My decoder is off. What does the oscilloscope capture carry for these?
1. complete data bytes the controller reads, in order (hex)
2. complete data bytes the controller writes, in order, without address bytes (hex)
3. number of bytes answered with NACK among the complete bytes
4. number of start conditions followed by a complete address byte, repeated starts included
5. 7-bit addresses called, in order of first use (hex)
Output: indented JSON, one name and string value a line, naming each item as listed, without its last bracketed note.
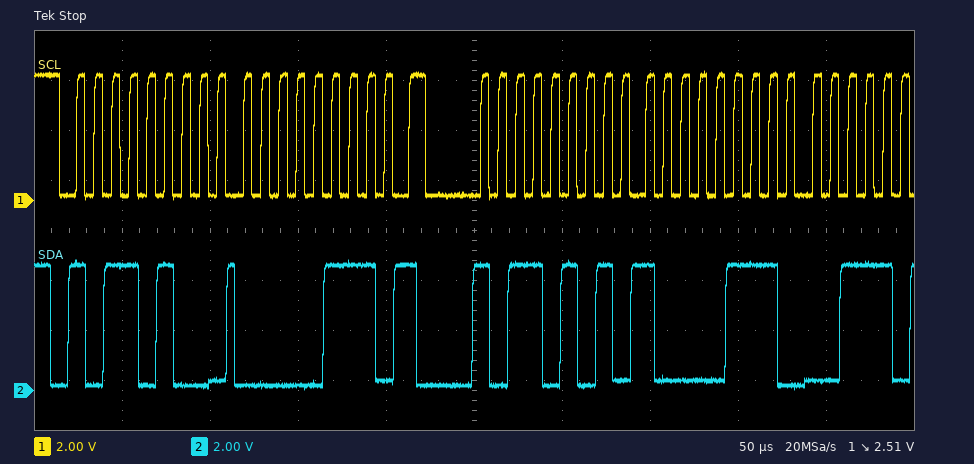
{
  "complete data bytes the controller reads, in order": "87",
  "complete data bytes the controller writes, in order, without address bytes": "07",
  "number of bytes answered with NACK among the complete bytes": "0",
  "number of start conditions followed by a complete address byte, repeated starts included": "2",
  "7-bit addresses called, in order of first use": "0x5A"
}
